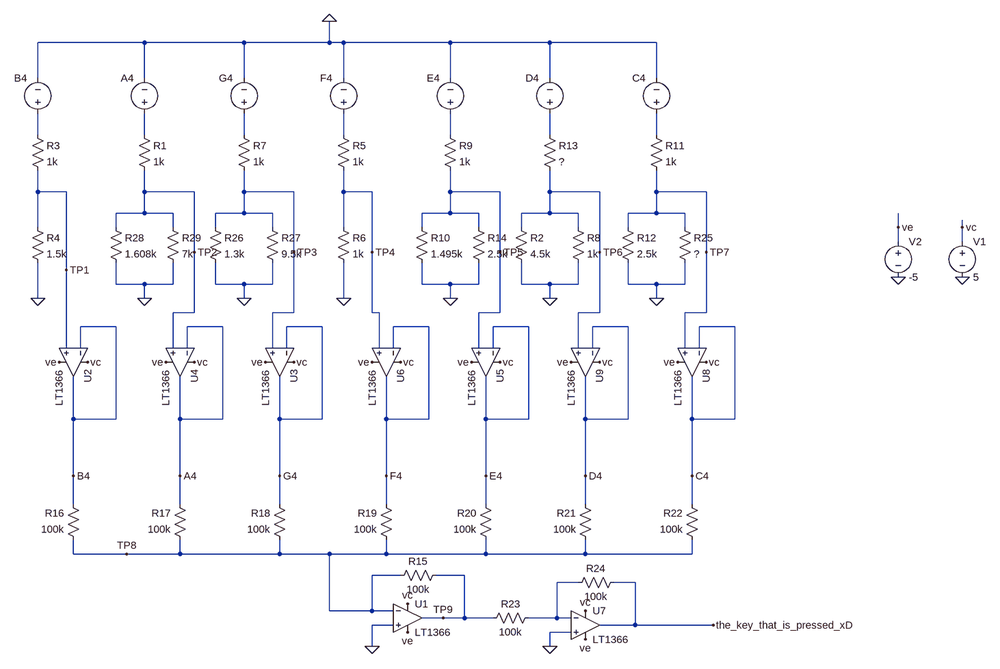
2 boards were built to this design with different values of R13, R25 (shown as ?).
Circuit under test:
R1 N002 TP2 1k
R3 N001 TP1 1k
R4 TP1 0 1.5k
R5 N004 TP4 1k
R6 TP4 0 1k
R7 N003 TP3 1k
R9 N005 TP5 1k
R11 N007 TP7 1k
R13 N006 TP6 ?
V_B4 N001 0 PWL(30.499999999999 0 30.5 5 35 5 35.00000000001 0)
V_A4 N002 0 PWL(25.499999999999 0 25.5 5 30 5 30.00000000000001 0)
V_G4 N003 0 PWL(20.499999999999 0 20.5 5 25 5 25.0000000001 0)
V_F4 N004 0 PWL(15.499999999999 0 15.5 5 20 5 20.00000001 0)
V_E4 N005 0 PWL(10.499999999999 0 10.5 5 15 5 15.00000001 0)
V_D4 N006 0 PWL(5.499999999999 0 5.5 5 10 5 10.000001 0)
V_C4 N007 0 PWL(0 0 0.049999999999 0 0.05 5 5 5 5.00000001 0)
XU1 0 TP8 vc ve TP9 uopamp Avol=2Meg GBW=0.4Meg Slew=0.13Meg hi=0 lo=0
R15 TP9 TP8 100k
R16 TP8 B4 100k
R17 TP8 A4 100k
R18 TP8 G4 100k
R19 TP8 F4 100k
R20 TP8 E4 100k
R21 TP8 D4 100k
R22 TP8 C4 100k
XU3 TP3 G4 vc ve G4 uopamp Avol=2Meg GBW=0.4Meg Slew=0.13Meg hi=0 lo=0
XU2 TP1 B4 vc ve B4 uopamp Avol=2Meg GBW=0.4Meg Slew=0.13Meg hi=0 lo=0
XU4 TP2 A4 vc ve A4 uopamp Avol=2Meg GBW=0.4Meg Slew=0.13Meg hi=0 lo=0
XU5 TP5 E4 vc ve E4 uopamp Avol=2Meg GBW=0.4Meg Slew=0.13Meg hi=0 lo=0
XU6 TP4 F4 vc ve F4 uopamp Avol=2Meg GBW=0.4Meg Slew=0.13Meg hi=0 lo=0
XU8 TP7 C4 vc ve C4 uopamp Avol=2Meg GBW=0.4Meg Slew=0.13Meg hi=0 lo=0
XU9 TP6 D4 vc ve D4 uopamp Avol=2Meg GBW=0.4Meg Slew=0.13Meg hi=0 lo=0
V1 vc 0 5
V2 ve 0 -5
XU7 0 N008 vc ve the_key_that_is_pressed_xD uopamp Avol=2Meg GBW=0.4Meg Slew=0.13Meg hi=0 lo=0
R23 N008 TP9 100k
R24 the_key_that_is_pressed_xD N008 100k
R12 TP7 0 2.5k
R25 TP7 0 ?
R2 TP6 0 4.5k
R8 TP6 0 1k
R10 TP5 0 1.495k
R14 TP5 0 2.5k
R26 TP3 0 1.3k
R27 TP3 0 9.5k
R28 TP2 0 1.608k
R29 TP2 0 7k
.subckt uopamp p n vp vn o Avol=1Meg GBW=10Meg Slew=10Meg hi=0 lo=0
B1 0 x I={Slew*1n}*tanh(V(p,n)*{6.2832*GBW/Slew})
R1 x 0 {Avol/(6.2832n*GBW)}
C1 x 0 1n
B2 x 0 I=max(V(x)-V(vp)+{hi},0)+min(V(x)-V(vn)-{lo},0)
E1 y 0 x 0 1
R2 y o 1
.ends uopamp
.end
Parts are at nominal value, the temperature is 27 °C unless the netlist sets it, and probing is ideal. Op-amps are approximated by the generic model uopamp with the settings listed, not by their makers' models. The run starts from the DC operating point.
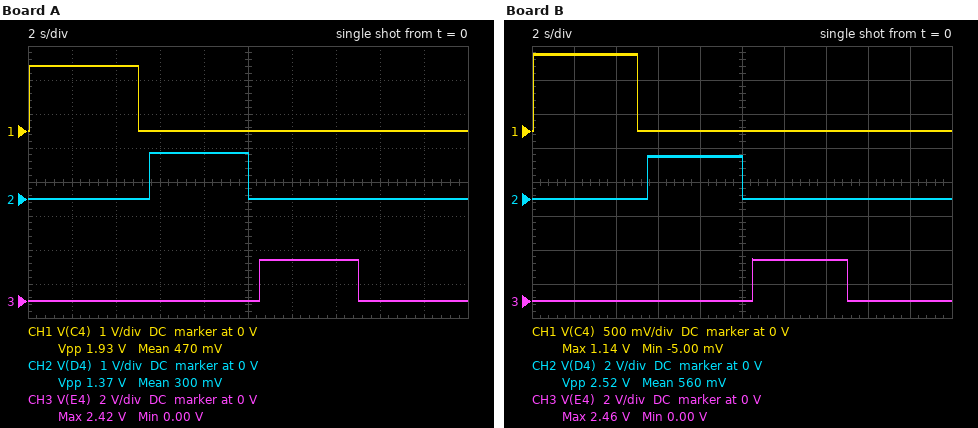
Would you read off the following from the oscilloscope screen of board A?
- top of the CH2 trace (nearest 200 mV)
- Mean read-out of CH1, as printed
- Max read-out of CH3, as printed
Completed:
1.4 V
470 mV
2.42 V
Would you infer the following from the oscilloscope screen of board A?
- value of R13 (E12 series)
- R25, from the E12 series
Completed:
2.2 kΩ
820 Ω
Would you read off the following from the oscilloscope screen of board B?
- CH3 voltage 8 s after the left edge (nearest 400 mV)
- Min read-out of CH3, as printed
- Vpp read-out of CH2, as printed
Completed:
0 V
0.00 V
2.52 V
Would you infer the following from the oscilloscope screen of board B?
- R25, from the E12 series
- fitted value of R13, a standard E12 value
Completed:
330 Ω
820 Ω
